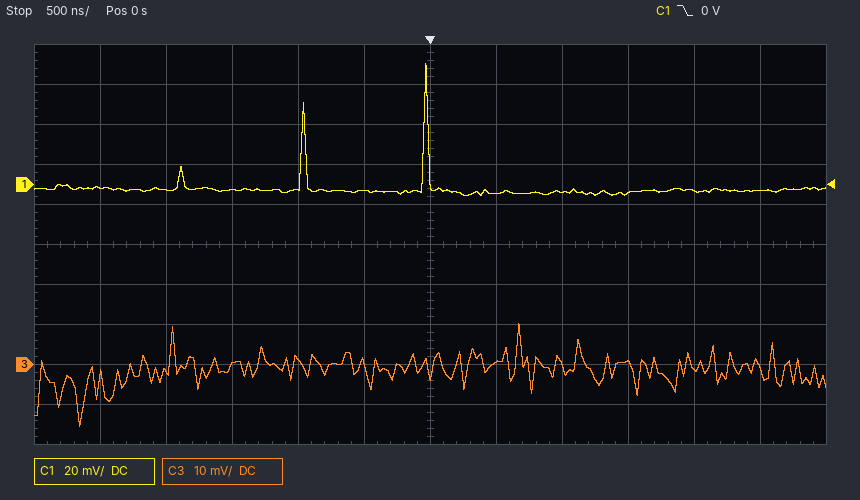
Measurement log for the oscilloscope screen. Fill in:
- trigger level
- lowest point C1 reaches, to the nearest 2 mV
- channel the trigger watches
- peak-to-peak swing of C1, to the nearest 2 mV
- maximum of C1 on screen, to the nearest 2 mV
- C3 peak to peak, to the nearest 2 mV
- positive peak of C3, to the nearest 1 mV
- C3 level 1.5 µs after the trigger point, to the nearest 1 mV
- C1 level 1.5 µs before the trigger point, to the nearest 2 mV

0 V
-6 mV
C1
66 mV
60 mV
26 mV
10 mV
0 mV
-2 mV
